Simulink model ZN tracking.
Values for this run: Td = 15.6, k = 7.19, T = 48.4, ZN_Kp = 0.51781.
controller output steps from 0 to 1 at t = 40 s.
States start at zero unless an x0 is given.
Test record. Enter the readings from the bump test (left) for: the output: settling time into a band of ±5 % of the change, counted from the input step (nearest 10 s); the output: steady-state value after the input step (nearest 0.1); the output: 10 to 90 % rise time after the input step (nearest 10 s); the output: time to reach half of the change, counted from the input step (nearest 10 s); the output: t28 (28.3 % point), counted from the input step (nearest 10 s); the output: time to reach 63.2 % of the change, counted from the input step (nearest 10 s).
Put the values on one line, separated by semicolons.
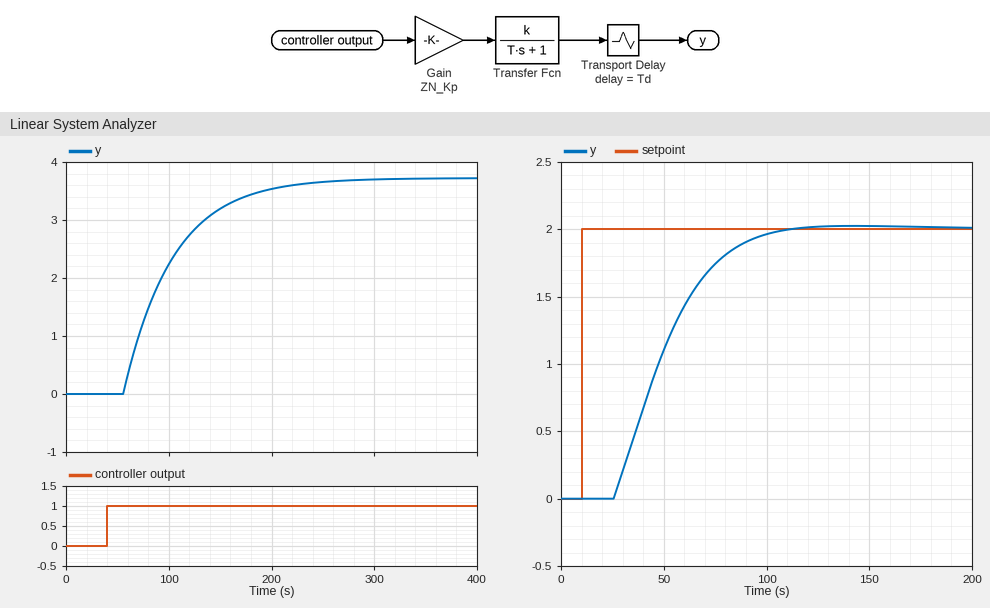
160 s; 3.7; 110 s; 50 s; 30 s; 60 s
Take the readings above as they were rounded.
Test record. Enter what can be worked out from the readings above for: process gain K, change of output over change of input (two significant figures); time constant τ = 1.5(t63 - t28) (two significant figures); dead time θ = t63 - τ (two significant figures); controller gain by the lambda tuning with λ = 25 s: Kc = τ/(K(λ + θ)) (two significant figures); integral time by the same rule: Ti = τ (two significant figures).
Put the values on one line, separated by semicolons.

3.7; 45 s; 15 s; 0.30; 45 s
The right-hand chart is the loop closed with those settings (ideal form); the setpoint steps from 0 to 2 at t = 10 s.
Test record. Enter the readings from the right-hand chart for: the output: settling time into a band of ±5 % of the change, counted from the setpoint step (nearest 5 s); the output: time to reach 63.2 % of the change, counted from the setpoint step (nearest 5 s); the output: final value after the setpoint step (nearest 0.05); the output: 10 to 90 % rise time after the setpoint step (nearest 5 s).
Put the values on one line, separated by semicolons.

80 s; 45 s; 2.00; 50 s
